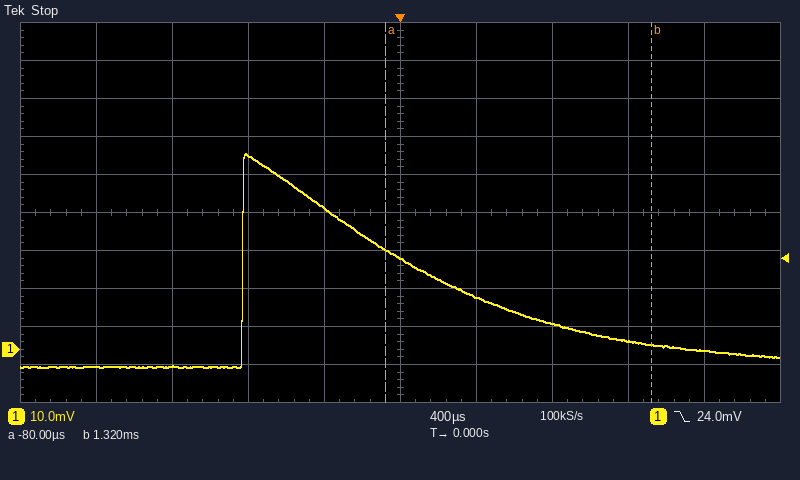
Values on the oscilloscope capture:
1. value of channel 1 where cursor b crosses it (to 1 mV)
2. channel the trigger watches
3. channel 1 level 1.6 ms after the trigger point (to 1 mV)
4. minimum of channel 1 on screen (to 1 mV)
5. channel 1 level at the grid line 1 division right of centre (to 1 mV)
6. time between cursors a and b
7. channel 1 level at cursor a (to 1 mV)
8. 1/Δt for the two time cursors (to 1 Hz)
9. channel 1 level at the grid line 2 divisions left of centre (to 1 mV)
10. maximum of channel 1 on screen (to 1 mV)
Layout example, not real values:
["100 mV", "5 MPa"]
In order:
["1 mV", "channel 1", "0 mV", "-5 mV", "14 mV", "1.40 ms", "26 mV", "714 Hz", "51 mV", "52 mV"]
